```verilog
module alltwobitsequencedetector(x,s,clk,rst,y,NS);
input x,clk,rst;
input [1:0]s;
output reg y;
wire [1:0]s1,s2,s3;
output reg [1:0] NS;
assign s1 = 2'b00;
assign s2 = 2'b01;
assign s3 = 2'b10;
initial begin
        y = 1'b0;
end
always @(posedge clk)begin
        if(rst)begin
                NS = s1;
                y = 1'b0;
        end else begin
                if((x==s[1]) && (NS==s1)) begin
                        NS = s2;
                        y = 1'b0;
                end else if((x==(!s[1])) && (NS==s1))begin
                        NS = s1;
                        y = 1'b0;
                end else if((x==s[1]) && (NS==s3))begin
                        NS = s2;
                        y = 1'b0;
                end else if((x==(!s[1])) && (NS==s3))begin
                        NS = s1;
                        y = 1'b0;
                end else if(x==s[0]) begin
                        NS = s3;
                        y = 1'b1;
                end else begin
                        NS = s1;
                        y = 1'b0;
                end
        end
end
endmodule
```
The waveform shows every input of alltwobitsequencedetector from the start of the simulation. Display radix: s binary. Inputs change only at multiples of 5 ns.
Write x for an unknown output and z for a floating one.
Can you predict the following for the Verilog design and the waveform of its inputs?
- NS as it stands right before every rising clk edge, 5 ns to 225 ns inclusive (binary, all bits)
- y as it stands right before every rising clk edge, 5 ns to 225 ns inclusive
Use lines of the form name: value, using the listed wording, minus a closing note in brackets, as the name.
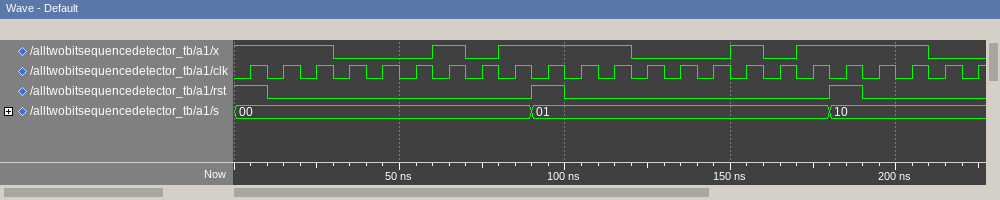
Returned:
NS as it stands right before every rising clk edge, 5 ns to 225 ns inclusive: x, 00, 00, 00, 01, 10, 01, 00, 01, 00, 00, 00, 00, 01, 00, 01, 10, 01, 10, 00, 01, 00, 00
y as it stands right before every rising clk edge, 5 ns to 225 ns inclusive: 0 0 0 0 0 1 0 0 0 0 0 0 0 0 0 0 1 0 1 0 0 0 0
